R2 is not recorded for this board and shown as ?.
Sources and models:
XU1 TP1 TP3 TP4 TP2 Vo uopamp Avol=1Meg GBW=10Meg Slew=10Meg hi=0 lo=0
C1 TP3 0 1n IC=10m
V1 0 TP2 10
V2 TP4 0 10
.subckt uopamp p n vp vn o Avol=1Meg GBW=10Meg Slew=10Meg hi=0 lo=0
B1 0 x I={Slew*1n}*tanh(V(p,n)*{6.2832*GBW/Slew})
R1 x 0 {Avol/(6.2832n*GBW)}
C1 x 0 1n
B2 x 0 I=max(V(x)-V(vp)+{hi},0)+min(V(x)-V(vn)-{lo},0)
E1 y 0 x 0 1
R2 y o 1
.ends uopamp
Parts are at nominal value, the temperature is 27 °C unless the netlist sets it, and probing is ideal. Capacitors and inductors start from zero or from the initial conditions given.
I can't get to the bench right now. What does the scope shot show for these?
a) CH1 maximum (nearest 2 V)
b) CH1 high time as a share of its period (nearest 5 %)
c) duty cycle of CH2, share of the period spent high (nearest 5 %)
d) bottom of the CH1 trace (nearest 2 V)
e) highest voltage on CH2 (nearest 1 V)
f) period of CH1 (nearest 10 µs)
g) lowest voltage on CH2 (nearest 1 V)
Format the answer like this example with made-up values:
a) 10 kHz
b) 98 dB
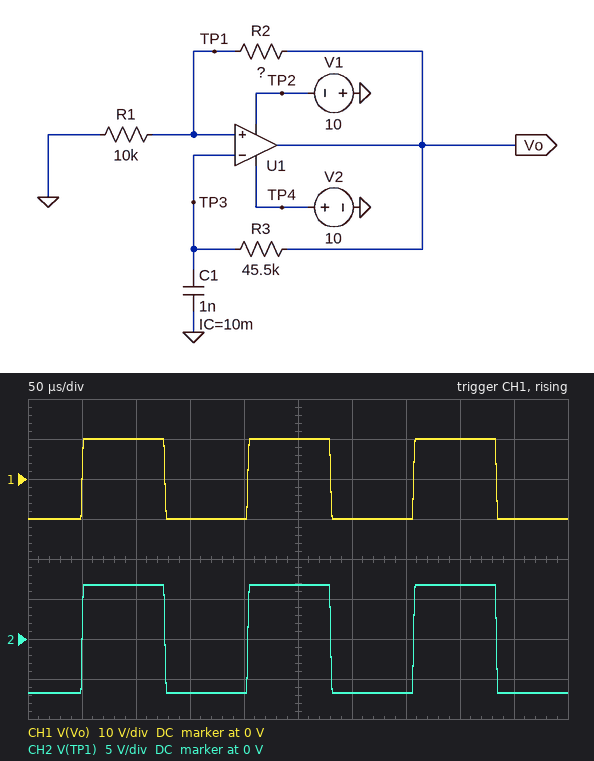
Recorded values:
a) 10 V
b) 50 %
c) 50 %
d) -10 V
e) 7 V
f) 150 µs
g) -7 V
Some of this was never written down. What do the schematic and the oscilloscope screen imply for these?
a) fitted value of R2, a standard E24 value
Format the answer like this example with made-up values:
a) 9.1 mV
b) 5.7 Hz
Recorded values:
a) 4.7 kΩ
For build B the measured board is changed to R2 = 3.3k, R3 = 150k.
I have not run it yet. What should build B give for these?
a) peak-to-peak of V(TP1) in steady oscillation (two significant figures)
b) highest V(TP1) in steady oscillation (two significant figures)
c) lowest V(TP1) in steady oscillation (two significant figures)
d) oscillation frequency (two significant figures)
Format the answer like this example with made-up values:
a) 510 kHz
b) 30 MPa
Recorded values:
a) 15 V
b) 7.5 V
c) -7.5 V
d) 1.7 kHz
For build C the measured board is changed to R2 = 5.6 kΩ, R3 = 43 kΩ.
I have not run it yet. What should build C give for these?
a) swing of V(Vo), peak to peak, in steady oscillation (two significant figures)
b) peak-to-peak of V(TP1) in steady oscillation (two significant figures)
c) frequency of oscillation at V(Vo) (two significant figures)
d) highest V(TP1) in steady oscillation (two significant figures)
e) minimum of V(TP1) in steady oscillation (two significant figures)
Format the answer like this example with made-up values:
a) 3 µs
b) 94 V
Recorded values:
a) 20 V
b) 13 V
c) 7.5 kHz
d) 6.4 V
e) -6.4 V
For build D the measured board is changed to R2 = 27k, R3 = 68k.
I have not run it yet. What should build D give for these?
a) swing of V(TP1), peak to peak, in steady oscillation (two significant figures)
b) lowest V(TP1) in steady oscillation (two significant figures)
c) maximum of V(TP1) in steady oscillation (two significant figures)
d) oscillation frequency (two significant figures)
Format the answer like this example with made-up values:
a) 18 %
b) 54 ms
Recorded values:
a) 5.4 V
b) -2.7 V
c) 2.7 V
d) 13 kHz
